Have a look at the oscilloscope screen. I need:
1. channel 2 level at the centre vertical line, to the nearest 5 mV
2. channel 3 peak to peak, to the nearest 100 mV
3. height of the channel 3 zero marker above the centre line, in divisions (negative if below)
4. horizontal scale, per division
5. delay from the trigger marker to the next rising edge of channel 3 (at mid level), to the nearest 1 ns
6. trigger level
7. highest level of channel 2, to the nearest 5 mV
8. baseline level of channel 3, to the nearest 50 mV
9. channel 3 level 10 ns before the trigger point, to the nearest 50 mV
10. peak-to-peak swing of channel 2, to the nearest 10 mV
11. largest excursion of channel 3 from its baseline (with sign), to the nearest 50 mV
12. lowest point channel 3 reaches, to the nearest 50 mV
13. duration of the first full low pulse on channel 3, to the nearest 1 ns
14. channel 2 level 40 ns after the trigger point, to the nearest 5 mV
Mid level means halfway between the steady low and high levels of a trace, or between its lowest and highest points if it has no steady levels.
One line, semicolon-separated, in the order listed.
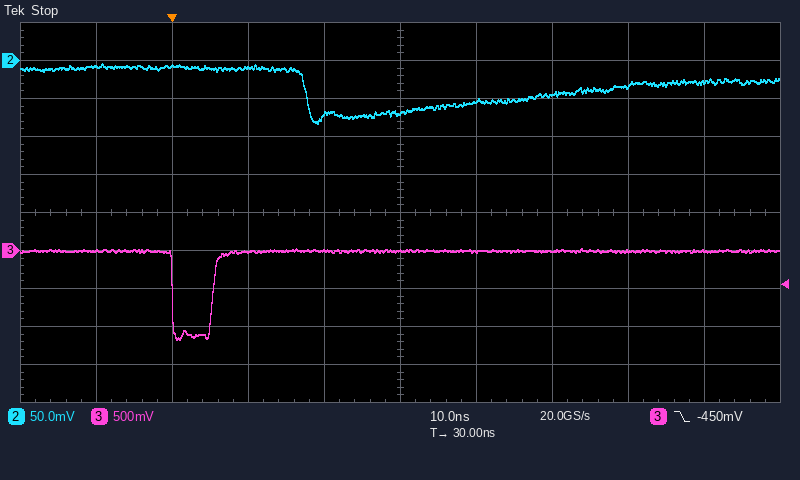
-70 mV; 1.20 V; -1.0 div; 10 ns; 5 ns; -450 mV; -5 mV; 0 mV; 0 mV; 80 mV; -1.15 V; -1.15 V; 5 ns; -55 mV
